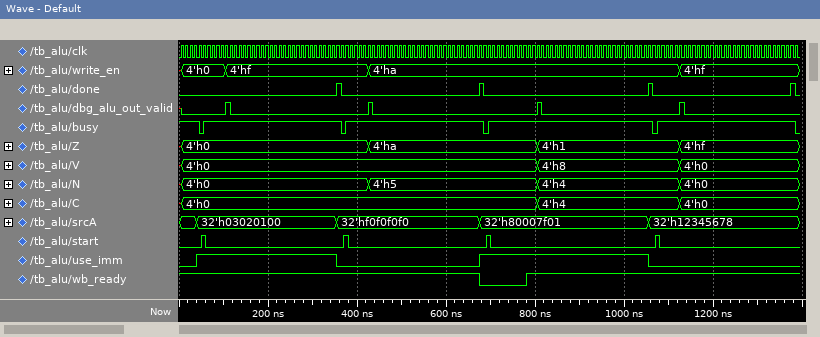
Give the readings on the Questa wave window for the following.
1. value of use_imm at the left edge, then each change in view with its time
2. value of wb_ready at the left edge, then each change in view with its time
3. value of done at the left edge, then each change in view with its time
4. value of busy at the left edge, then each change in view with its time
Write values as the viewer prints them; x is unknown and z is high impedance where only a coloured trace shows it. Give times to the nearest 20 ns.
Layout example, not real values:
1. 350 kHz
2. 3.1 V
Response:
1. 0, 1 at 40 ns, 0 at 360 ns, 1 at 680 ns, 0 at 1060 ns
2. 1, 0 at 680 ns, 1 at 780 ns
3. 0, 1 at 360 ns, 0 at 360 ns, 1 at 680 ns, 0 at 680 ns, 1 at 1060 ns, 0 at 1060 ns, 1 at 1380 ns, 0 at 1380 ns
4. 1, 0 at 40 ns, 1 at 60 ns, 0 at 360 ns, 1 at 380 ns, 0 at 680 ns, 1 at 700 ns, 0 at 1060 ns, 1 at 1080 ns, 0 at 1380 ns
